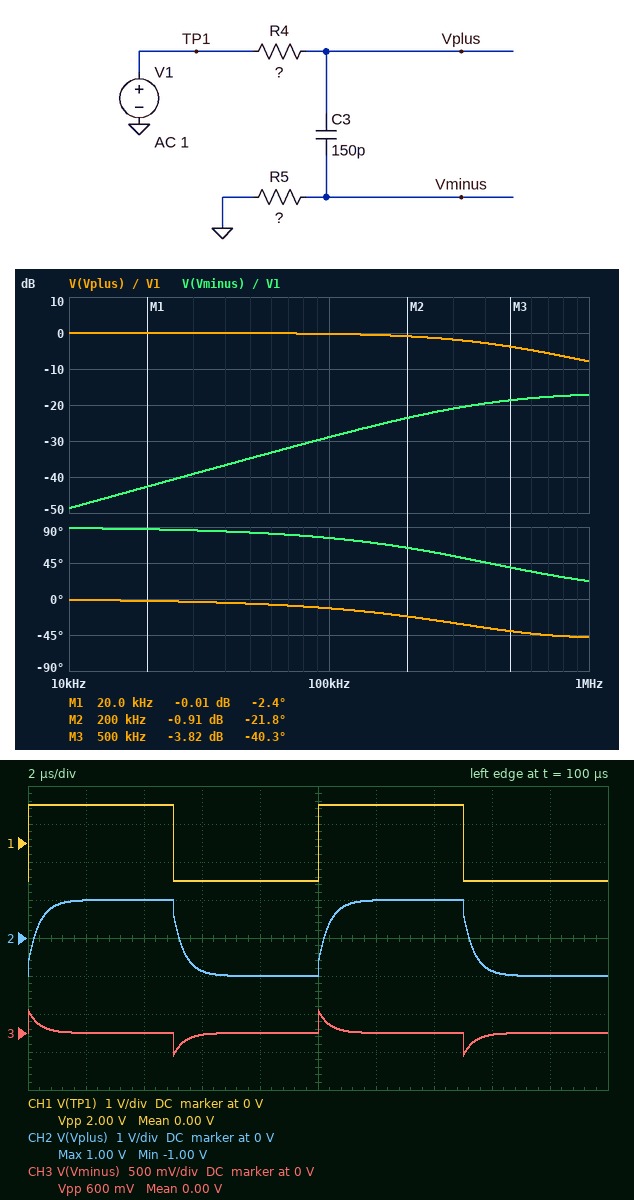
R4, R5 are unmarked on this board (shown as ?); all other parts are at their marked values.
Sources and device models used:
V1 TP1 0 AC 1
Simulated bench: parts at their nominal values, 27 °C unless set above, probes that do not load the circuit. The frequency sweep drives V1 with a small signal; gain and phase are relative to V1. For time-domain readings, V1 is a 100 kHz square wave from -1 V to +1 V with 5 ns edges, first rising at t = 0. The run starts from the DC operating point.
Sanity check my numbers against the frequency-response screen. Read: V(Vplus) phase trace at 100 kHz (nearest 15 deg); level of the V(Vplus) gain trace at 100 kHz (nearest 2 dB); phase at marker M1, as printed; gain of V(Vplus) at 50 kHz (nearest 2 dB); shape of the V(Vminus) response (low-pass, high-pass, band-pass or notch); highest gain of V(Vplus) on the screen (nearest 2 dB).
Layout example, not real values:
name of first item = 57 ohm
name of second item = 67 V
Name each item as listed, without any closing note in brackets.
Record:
V(Vplus) phase trace at 100 kHz = -15 deg
level of the V(Vplus) gain trace at 100 kHz = 0 dB
phase at marker M1, as printed = -2.4 deg
gain of V(Vplus) at 50 kHz = 0 dB
shape of the V(Vminus) response = high-pass
highest gain of V(Vplus) on the screen = 0 dB
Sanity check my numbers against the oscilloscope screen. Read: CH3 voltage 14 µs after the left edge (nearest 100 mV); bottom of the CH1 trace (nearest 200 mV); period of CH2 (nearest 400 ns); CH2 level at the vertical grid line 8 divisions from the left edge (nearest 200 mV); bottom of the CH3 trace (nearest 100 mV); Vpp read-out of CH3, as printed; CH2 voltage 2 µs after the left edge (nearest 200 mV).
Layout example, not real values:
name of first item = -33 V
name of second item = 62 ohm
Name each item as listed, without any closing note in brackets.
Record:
CH3 voltage 14 µs after the left edge = 0 V
bottom of the CH1 trace = -1.0 V
period of CH2 = 10.0 µs
CH2 level at the vertical grid line 8 divisions from the left edge = -800 mV
bottom of the CH3 trace = -300 mV
Vpp read-out of CH3, as printed = 600 mV
CH2 voltage 2 µs after the left edge = 1.0 V
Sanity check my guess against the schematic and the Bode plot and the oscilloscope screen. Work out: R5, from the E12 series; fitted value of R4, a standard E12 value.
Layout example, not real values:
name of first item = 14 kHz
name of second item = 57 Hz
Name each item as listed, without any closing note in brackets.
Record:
R5, from the E12 series = 390 Ω
fitted value of R4, a standard E12 value = 2.2 kΩ
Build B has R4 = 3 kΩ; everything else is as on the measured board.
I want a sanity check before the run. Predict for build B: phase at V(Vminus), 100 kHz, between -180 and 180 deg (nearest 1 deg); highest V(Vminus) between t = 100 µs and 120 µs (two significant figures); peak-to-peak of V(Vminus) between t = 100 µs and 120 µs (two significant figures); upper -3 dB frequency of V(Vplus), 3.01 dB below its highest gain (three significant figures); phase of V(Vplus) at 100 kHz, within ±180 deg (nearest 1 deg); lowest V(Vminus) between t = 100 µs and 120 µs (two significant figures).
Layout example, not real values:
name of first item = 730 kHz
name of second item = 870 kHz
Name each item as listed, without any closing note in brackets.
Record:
phase at V(Vminus), 100 kHz, between -180 and 180 deg = 72 deg
highest V(Vminus) between t = 100 µs and 120 µs = 230 mV
peak-to-peak of V(Vminus) between t = 100 µs and 120 µs = 460 mV
upper -3 dB frequency of V(Vplus), 3.01 dB below its highest gain = 317 kHz
phase of V(Vplus) at 100 kHz, within ±180 deg = -16 deg
lowest V(Vminus) between t = 100 µs and 120 µs = -230 mV
